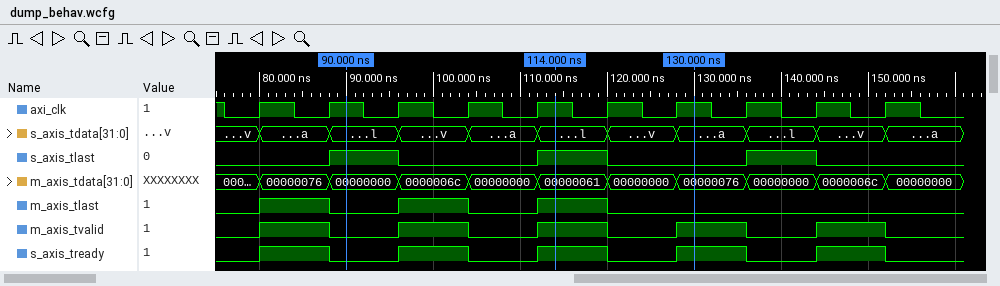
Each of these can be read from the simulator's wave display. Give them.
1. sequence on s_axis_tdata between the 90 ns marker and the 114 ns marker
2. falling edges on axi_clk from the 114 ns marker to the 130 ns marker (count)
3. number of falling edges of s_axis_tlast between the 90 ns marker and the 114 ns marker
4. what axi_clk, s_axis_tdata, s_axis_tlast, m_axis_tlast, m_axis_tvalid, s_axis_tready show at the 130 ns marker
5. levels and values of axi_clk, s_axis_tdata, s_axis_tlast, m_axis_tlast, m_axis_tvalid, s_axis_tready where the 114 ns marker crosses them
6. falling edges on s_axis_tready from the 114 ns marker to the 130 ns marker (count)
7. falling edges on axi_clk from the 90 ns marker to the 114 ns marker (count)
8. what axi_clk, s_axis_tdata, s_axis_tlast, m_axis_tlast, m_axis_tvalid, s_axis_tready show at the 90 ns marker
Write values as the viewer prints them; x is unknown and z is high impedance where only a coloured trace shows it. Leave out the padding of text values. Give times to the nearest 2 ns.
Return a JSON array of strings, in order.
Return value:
["l, v, a, l", "2", "1", "axi_clk=1, s_axis_tdata=a, s_axis_tlast=0, m_axis_tlast=0, m_axis_tvalid=1, s_axis_tready=1", "axi_clk=1, s_axis_tdata=l, s_axis_tlast=1, m_axis_tlast=1, m_axis_tvalid=1, s_axis_tready=1", "1", "3", "axi_clk=1, s_axis_tdata=l, s_axis_tlast=1, m_axis_tlast=0, m_axis_tvalid=0, s_axis_tready=0"]
